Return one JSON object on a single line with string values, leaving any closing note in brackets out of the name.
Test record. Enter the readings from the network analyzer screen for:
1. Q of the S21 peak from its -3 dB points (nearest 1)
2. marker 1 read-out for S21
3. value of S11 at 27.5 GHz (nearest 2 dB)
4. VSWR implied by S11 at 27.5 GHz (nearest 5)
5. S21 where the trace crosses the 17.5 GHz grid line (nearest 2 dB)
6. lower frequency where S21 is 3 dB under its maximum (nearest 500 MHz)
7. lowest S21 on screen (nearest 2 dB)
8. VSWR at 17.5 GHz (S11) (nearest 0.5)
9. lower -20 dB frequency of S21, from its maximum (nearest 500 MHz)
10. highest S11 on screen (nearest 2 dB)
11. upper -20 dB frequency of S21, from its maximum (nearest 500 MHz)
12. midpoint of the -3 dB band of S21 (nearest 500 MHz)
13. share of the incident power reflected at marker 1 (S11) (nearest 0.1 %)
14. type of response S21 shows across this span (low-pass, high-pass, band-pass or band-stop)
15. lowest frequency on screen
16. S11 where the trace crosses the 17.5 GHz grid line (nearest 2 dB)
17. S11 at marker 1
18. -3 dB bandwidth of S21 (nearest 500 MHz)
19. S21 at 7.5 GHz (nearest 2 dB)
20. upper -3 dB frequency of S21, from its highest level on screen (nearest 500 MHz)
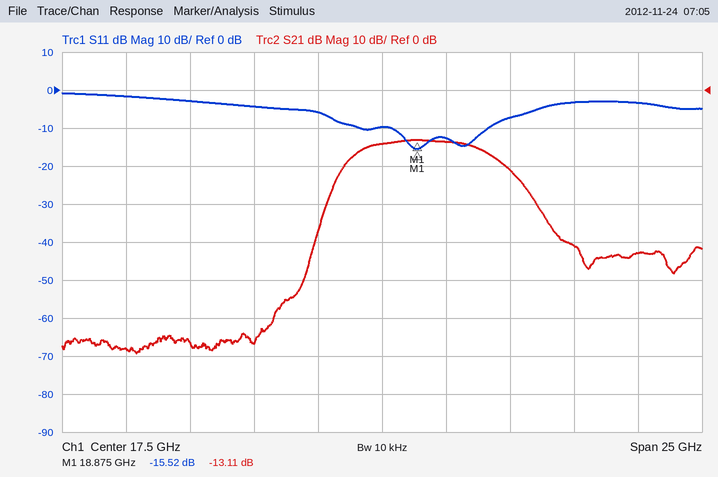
{"Q of the S21 peak from its -3 dB points": "4", "marker 1 read-out for S21": "-13.11 dB", "value of S11 at 27.5 GHz": "-4 dB", "VSWR implied by S11 at 27.5 GHz": "5", "S21 where the trace crosses the 17.5 GHz grid line": "-14 dB", "lower frequency where S21 is 3 dB under its maximum": "16.5 GHz", "lowest S21 on screen": "-70 dB", "VSWR at 17.5 GHz (S11)": "2.0", "lower -20 dB frequency of S21, from its maximum": "15.0 GHz", "highest S11 on screen": "0 dB", "upper -20 dB frequency of S21, from its maximum": "24.0 GHz", "midpoint of the -3 dB band of S21": "19.0 GHz", "share of the incident power reflected at marker 1 (S11)": "2.8 %", "type of response S21 shows across this span": "band-pass", "lowest frequency on screen": "5 GHz", "S11 where the trace crosses the 17.5 GHz grid line": "-10 dB", "S11 at marker 1": "-15.52 dB", "-3 dB bandwidth of S21": "5.0 GHz", "S21 at 7.5 GHz": "-68 dB", "upper -3 dB frequency of S21, from its highest level on screen": "21.5 GHz"}
